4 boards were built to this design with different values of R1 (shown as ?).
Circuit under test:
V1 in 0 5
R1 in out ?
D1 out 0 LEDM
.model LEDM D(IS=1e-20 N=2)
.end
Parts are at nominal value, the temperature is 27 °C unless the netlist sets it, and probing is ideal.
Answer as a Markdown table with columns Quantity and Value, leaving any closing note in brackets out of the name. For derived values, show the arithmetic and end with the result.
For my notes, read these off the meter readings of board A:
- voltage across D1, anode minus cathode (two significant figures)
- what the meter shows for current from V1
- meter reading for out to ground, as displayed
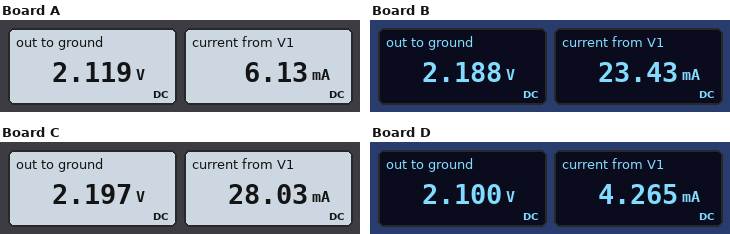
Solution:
| Quantity | Value |
|---|---|
| voltage across D1, anode minus cathode | 2.119 V = 2.1 V |
| what the meter shows for current from V1 | 6.13 mA |
| meter reading for out to ground, as displayed | 2.119 V |
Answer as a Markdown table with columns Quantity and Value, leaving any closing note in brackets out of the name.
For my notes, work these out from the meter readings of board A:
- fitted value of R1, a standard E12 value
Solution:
| Quantity | Value |
|---|---|
| fitted value of R1, a standard E12 value | 470 Ω |
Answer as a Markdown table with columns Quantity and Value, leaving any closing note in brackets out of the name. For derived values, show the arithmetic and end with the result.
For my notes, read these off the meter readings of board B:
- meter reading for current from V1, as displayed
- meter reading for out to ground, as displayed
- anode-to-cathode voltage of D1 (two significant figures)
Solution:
| Quantity | Value |
|---|---|
| meter reading for current from V1, as displayed | 23.43 mA |
| meter reading for out to ground, as displayed | 2.188 V |
| anode-to-cathode voltage of D1 | 2.188 V = 2.2 V |
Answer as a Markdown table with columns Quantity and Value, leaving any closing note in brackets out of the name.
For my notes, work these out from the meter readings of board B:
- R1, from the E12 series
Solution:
| Quantity | Value |
|---|---|
| R1, from the E12 series | 120 Ω |
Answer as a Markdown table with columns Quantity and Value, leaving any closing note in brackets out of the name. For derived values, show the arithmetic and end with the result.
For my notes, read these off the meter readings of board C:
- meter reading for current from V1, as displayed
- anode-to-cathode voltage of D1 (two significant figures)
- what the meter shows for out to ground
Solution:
| Quantity | Value |
|---|---|
| meter reading for current from V1, as displayed | 28.03 mA |
| anode-to-cathode voltage of D1 | 2.197 V = 2.2 V |
| what the meter shows for out to ground | 2.197 V |
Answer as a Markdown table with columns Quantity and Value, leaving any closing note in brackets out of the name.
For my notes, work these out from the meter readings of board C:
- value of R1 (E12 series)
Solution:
| Quantity | Value |
|---|---|
| value of R1 | 100 Ω |
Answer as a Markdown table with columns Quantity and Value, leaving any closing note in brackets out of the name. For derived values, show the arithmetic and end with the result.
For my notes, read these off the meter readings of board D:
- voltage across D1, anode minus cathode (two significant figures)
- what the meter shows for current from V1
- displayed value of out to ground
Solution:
| Quantity | Value |
|---|---|
| voltage across D1, anode minus cathode | 2.1 V = 2.1 V |
| what the meter shows for current from V1 | 4.265 mA |
| displayed value of out to ground | 2.100 V |
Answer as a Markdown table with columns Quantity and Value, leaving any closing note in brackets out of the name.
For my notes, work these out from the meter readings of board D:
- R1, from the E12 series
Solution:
| Quantity | Value |
|---|---|
| R1, from the E12 series | 680 Ω |
